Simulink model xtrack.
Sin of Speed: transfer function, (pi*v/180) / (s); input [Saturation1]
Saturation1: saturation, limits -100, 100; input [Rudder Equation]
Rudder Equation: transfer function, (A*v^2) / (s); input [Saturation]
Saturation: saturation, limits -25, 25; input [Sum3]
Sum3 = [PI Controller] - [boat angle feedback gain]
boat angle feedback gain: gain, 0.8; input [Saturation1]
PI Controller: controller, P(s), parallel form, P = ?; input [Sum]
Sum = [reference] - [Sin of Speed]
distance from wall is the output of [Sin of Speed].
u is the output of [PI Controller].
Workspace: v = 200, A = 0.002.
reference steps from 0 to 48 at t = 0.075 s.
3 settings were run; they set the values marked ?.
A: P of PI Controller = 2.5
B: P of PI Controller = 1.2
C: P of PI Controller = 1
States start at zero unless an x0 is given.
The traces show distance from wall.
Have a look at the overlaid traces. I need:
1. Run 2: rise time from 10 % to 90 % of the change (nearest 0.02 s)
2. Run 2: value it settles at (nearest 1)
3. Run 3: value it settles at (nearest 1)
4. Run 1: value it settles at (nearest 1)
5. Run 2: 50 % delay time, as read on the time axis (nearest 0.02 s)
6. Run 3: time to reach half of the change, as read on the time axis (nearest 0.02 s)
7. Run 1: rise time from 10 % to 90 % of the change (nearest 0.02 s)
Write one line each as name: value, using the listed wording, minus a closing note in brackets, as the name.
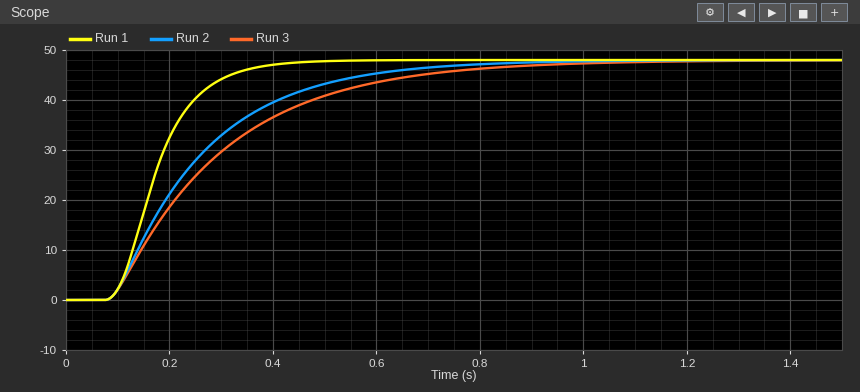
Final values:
Run 2: rise time from 10 % to 90 % of the change: 0.38 s
Run 2: value it settles at: 48
Run 3: value it settles at: 48
Run 1: value it settles at: 48
Run 2: 50 % delay time, as read on the time axis: 0.22 s
Run 3: time to reach half of the change, as read on the time axis: 0.24 s
Run 1: rise time from 10 % to 90 % of the change: 0.18 s
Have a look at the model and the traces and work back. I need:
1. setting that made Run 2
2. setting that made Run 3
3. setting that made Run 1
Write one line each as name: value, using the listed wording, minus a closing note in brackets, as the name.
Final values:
setting that made Run 2: B
setting that made Run 3: C
setting that made Run 1: A
